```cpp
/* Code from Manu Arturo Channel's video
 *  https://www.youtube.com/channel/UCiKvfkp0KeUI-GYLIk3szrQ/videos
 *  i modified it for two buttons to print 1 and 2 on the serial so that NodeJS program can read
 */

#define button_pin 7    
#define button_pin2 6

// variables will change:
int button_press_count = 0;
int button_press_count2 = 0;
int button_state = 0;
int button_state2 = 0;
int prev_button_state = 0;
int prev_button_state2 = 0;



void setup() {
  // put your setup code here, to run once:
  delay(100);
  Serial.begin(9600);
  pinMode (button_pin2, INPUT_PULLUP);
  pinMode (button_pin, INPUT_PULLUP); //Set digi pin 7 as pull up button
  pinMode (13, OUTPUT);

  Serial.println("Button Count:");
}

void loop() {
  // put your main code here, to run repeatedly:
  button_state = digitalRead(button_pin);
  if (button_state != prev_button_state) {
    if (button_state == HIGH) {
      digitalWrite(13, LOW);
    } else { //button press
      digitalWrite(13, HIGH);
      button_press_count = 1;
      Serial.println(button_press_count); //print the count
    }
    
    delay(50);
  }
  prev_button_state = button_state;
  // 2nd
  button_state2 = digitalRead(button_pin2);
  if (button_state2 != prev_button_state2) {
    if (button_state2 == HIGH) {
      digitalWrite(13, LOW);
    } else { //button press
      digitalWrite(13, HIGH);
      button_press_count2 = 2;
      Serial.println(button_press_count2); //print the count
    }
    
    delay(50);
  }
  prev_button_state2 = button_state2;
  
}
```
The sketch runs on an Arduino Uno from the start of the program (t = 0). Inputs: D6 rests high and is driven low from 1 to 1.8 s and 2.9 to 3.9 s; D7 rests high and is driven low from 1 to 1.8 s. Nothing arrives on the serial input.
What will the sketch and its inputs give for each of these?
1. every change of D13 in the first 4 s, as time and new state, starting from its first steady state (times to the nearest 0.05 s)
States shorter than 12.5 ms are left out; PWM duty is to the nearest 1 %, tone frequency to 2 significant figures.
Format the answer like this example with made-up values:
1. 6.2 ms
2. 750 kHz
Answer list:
1. 0.1 s low; 1 s high; 1.8 s low; 2.9 s high; 3.9 s low
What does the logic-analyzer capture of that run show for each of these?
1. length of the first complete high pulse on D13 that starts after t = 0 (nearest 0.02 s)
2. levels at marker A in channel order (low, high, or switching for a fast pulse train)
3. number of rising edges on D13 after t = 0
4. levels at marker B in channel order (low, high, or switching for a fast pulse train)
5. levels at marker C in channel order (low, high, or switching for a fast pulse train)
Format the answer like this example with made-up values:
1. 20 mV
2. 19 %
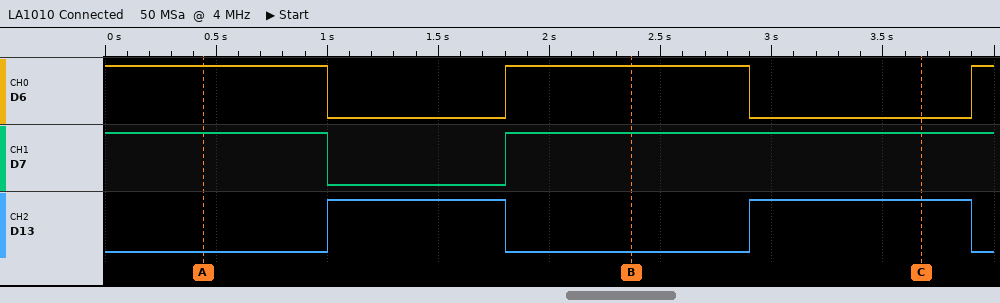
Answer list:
1. 0.80 s
2. D6 high, D7 high, D13 low
3. 2
4. D6 high, D7 high, D13 low
5. D6 low, D7 high, D13 high
